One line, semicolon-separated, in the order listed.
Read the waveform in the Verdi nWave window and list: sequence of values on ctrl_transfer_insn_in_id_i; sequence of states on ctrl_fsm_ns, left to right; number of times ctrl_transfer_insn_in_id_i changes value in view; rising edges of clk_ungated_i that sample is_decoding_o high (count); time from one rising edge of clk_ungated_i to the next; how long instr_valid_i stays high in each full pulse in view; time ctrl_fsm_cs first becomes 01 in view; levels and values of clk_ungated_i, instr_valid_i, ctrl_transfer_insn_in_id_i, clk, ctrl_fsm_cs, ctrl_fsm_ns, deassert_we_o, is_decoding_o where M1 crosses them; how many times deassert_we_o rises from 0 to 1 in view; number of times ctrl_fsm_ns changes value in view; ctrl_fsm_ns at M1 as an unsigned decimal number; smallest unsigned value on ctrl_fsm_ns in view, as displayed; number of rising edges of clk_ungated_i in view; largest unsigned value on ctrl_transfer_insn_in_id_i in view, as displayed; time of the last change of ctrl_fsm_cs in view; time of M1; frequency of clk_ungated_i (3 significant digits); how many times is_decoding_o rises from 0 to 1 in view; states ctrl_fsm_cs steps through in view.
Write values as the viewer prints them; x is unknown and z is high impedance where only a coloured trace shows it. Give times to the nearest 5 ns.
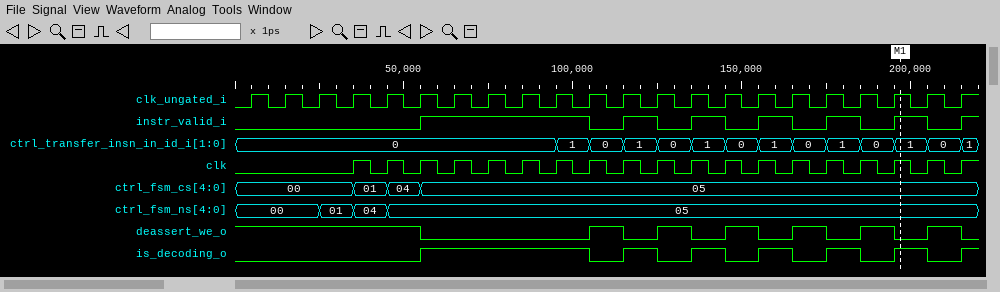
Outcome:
0, 1, 0, 1, 0, 1, 0, 1, 0, 1, 0, 1, 0, 1; 00, 01, 04, 05; 13; 10; 10 ns; 50 ns, 10 ns, 10 ns, 10 ns, 10 ns, 10 ns; 35 ns; clk_ungated_i=1, instr_valid_i=1, ctrl_transfer_insn_in_id_i=1, clk=1, ctrl_fsm_cs=05, ctrl_fsm_ns=05, deassert_we_o=0, is_decoding_o=1; 6; 3; 5; 00; 22; 1; 55 ns; 195 ns; 100 MHz; 7; 00, 01, 04, 05
